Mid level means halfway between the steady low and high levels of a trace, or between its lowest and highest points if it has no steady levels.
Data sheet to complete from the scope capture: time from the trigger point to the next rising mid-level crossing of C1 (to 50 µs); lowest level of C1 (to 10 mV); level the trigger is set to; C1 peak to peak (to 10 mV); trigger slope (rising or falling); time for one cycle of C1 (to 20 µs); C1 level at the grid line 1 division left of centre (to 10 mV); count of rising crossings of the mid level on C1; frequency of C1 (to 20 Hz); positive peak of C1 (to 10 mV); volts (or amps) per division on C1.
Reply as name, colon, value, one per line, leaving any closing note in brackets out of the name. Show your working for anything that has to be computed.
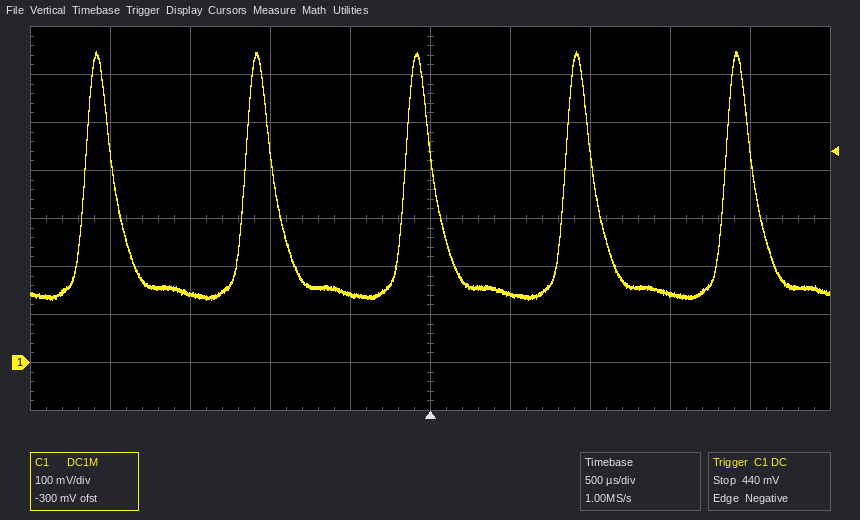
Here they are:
time from the trigger point to the next rising mid-level crossing of C1: 850 µs
lowest level of C1: 130 mV
level the trigger is set to: 440 mV
C1 peak to peak: 650 mV − (130 mV) = 520 mV
trigger slope: falling
time for one cycle of C1: 1.00 ms
C1 level at the grid line 1 division left of centre: 140 mV
count of rising crossings of the mid level on C1: 5
frequency of C1: 1 / 1.00 ms ≈ 1.00 kHz
positive peak of C1: 650 mV
volts (or amps) per division on C1: 100 mV
